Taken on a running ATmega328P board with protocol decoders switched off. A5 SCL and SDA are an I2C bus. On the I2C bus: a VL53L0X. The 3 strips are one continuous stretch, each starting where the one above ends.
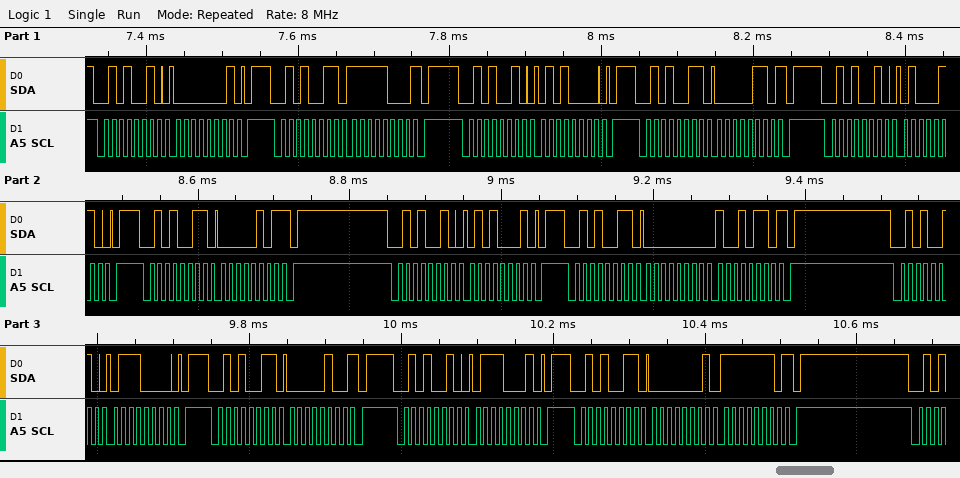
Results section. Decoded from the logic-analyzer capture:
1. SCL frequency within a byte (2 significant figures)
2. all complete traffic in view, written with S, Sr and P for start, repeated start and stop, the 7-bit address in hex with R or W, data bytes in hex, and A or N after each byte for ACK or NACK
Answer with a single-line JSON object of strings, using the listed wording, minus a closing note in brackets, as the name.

{"SCL frequency within a byte": "100 kHz", "all complete traffic in view, written with S, Sr and P for start, repeated start and stop, the 7-bit address in hex with R or W, data bytes in hex, and A or N after each byte for ACK or NACK": "S 29W A 01 A P S 29R A F8 N P S 29W A 50 A P S 29R A 06 N P S 29W A 46 A P S 29R A 05 N P S 29W A 51 A P S 29R A 00 A 96 N P S 29W A 70 A P S 29R A 04 N P S 29W A 71 A P S 29R A 01 A FE N P"}
